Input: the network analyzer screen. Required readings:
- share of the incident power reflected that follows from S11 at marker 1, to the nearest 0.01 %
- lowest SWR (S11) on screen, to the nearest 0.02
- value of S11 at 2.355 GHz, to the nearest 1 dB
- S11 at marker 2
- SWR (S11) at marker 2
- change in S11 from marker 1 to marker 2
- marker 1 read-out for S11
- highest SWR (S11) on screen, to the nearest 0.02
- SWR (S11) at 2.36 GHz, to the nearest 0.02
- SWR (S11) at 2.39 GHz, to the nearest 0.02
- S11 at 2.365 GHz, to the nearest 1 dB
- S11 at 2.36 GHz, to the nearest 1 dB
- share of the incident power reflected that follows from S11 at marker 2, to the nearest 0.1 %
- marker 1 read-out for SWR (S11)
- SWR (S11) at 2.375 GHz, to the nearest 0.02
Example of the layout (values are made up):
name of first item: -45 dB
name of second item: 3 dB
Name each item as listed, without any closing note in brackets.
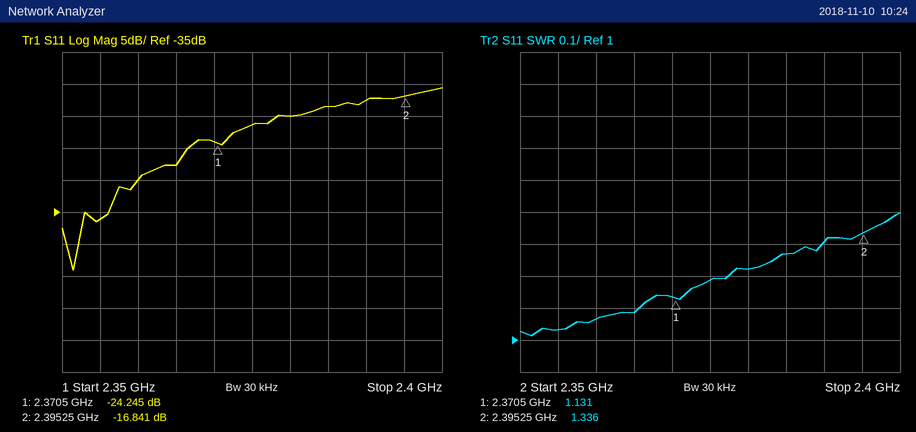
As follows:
share of the incident power reflected that follows from S11 at marker 1, to the nearest 0.01 %: 0.38 %
lowest SWR (S11) on screen, to the nearest 0.02: 1.02
value of S11 at 2.355 GHz, to the nearest 1 dB: -36 dB
S11 at marker 2: -16.841 dB
SWR (S11) at marker 2: 1.336
change in S11 from marker 1 to marker 2: 7.404 dB
marker 1 read-out for S11: -24.245 dB
highest SWR (S11) on screen, to the nearest 0.02: 1.40
SWR (S11) at 2.36 GHz, to the nearest 0.02: 1.06
SWR (S11) at 2.39 GHz, to the nearest 0.02: 1.30
S11 at 2.365 GHz, to the nearest 1 dB: -28 dB
S11 at 2.36 GHz, to the nearest 1 dB: -30 dB
share of the incident power reflected that follows from S11 at marker 2, to the nearest 0.1 %: 2.1 %
marker 1 read-out for SWR: 1.131
SWR (S11) at 2.375 GHz, to the nearest 0.02: 1.18
